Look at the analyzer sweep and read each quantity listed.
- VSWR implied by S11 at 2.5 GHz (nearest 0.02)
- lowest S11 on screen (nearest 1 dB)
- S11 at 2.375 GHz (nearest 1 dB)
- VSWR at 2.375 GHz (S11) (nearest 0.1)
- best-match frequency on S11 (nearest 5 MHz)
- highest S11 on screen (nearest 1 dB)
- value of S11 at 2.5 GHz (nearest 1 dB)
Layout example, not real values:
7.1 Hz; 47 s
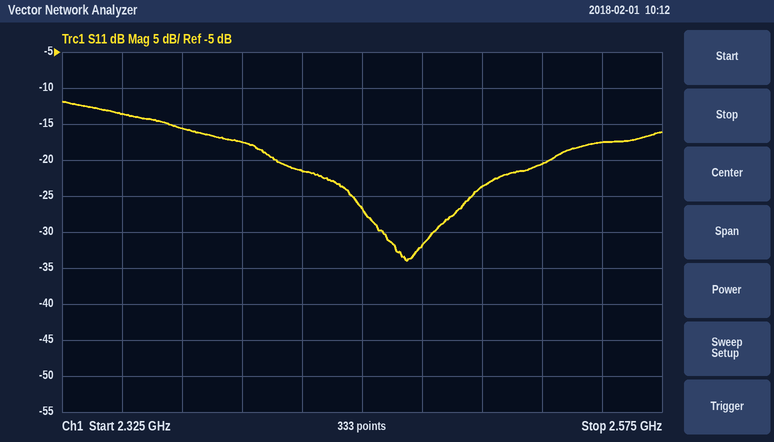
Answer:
1.14; -34 dB; -16 dB; 1.4; 2.470 GHz; -12 dB; -24 dB
